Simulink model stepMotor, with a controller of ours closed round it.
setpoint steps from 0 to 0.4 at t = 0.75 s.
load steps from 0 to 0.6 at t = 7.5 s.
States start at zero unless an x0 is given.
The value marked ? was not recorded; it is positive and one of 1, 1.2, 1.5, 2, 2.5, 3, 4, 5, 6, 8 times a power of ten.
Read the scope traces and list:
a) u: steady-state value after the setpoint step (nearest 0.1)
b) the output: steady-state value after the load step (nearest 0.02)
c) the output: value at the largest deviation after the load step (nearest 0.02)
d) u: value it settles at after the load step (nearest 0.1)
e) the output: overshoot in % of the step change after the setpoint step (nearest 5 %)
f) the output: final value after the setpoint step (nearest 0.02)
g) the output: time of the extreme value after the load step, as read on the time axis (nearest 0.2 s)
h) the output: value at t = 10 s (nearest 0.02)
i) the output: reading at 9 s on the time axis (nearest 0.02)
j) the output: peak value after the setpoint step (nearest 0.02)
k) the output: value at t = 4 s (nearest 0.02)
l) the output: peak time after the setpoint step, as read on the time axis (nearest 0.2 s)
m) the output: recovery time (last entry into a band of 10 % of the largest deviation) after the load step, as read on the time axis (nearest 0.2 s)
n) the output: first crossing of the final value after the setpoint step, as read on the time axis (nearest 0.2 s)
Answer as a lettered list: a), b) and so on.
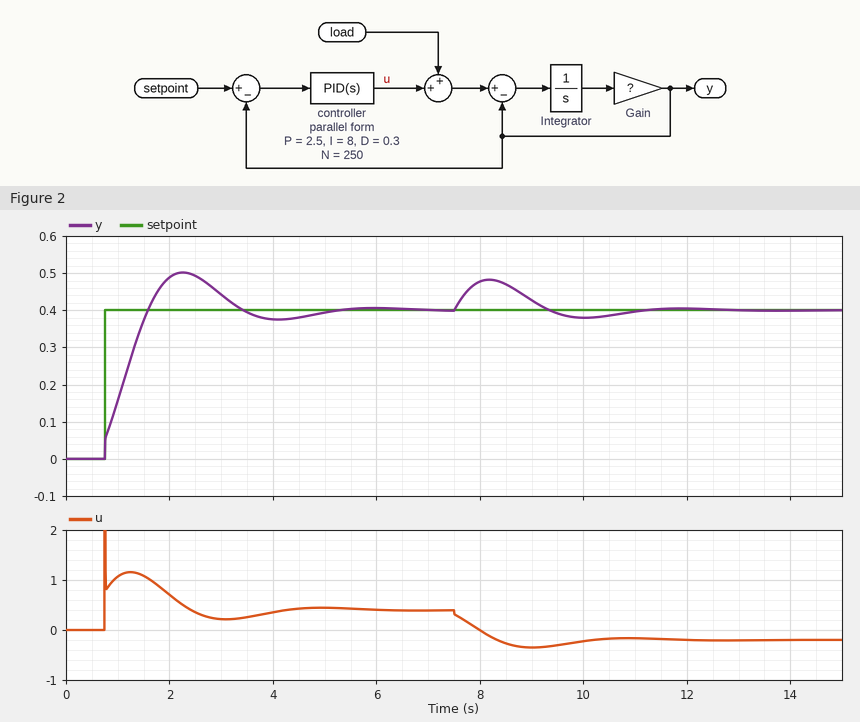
a) 0.4
b) 0.40
c) 0.48
d) -0.2
e) 25 %
f) 0.40
g) 8.2 s
h) 0.38
i) 0.42
j) 0.50
k) 0.38
l) 2.2 s
m) 10.8 s
n) 1.6 s
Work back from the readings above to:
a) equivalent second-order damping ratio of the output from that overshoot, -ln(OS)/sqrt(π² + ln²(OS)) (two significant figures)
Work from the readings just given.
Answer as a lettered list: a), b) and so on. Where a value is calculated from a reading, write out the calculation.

a) ln(0.25) = -1.386; 1.386 / sqrt(9.870 + 1.922) = 0.40
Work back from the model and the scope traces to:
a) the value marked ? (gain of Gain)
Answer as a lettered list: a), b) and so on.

a) 0.5
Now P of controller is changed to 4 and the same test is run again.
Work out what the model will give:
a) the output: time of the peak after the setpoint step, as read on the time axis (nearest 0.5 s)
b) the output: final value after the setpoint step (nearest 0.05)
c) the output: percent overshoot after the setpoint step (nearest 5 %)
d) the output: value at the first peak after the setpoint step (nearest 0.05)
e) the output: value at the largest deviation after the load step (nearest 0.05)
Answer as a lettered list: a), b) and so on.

a) 2.0 s
b) 0.40
c) 15 %
d) 0.45
e) 0.45
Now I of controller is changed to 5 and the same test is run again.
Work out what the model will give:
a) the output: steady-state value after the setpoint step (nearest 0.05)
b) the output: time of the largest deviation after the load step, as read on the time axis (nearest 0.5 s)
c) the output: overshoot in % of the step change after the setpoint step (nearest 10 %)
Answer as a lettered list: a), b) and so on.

a) 0.40
b) 8.5 s
c) 20 %
